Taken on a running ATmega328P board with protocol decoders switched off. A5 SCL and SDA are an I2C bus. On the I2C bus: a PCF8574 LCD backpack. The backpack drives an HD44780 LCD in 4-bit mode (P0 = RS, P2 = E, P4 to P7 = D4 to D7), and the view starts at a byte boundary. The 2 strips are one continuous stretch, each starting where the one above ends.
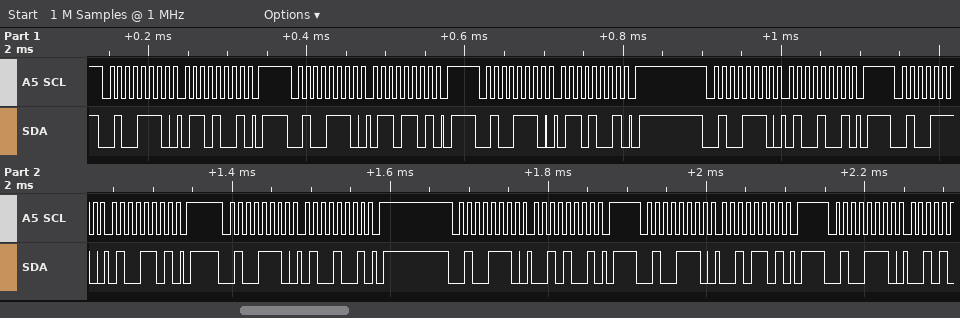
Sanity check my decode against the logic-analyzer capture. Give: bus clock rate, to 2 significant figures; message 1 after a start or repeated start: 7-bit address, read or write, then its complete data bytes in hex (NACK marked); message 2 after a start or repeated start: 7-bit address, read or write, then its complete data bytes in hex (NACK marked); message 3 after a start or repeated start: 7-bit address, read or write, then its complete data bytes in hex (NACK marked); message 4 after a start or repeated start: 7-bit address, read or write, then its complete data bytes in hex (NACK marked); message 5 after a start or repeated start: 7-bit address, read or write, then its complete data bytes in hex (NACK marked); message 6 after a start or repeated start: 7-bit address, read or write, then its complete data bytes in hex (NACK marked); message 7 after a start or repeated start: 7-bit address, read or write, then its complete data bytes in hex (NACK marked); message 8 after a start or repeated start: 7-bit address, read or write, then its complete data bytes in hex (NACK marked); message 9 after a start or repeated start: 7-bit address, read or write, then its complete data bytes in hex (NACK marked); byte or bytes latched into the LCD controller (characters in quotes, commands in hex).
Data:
100 kHz
0x27 write: 69
0x27 write: 6D
0x27 write: 69
0x27 write: 49
0x27 write: 4D
0x27 write: 49
0x27 write: 29
0x27 write: 2D
0x27 write
'd'
